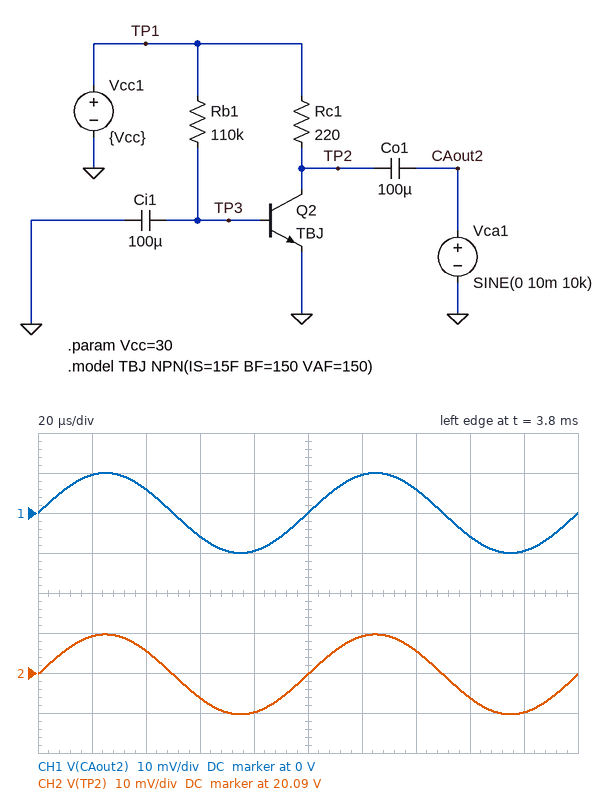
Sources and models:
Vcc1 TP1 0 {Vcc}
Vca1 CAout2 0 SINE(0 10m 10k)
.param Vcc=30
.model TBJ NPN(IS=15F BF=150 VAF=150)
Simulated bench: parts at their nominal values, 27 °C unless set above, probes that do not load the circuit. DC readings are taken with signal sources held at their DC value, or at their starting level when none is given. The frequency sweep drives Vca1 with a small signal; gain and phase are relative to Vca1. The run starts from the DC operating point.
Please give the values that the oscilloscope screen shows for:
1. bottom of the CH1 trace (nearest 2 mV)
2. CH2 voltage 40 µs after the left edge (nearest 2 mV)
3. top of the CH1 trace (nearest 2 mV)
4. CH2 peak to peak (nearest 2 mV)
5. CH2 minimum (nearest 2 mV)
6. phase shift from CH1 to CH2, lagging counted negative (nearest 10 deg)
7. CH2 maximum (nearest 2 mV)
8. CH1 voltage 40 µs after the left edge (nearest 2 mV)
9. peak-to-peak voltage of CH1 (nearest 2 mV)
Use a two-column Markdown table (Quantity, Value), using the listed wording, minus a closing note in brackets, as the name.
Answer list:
| Quantity | Value |
|---|---|
| bottom of the CH1 trace | -10 mV |
| CH2 voltage 40 µs after the left edge | 20.096 V |
| top of the CH1 trace | 10 mV |
| CH2 peak to peak | 20 mV |
| CH2 minimum | 20.080 V |
| phase shift from CH1 to CH2, lagging counted negative | 0 deg |
| CH2 maximum | 20.100 V |
| CH1 voltage 40 µs after the left edge | 6 mV |
| peak-to-peak voltage of CH1 | 20 mV |
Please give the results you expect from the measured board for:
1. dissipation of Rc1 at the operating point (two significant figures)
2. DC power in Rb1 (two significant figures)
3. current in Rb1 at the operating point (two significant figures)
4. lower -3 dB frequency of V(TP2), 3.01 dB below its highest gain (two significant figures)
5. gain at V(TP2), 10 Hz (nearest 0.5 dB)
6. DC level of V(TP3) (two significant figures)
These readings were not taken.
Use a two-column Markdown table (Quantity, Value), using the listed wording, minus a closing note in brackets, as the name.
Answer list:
| Quantity | Value |
|---|---|
| dissipation of Rc1 at the operating point | 450 mW |
| DC power in Rb1 | 7.8 mW |
| current in Rb1 at the operating point | 270 µA |
| lower -3 dB frequency of V(TP2), 3.01 dB below its highest gain | 7.7 Hz |
| gain at V(TP2), 10 Hz | -2.0 dB |
| DC level of V(TP3) | 740 mV |
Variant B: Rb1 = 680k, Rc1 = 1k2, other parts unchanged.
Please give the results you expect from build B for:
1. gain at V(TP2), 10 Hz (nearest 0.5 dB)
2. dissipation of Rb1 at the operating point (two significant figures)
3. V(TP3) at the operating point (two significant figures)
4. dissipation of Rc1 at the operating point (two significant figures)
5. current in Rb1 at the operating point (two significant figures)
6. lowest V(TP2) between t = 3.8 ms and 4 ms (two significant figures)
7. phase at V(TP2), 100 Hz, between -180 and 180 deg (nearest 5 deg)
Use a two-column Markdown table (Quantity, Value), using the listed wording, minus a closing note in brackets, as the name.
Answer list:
| Quantity | Value |
|---|---|
| gain at V(TP2), 10 Hz | 0 dB |
| dissipation of Rb1 at the operating point | 1.3 mW |
| V(TP3) at the operating point | 690 mV |
| dissipation of Rc1 at the operating point | 65 mW |
| current in Rb1 at the operating point | 43 µA |
| lowest V(TP2) between t = 3.8 ms and 4 ms | 21 V |
| phase at V(TP2), 100 Hz, between -180 and 180 deg | 0 deg |
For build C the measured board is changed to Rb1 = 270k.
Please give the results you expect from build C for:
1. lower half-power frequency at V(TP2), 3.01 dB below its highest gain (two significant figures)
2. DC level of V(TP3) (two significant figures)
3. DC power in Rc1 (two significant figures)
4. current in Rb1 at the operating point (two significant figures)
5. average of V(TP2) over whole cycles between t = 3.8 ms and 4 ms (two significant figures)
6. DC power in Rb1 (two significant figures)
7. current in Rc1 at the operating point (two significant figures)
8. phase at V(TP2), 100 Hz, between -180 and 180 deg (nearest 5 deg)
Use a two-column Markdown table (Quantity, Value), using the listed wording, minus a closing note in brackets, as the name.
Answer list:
| Quantity | Value |
|---|---|
| lower half-power frequency at V(TP2), 3.01 dB below its highest gain | 7.4 Hz |
| DC level of V(TP3) | 720 mV |
| DC power in Rc1 | 79 mW |
| current in Rb1 at the operating point | 110 µA |
| average of V(TP2) over whole cycles between t = 3.8 ms and 4 ms | 26 V |
| DC power in Rb1 | 3.2 mW |
| current in Rc1 at the operating point | 19 mA |
| phase at V(TP2), 100 Hz, between -180 and 180 deg | 5 deg |
